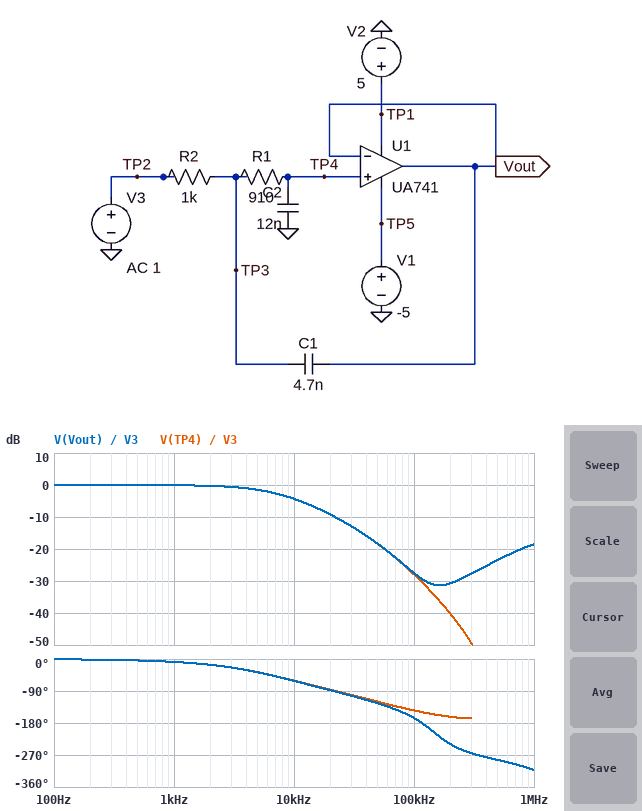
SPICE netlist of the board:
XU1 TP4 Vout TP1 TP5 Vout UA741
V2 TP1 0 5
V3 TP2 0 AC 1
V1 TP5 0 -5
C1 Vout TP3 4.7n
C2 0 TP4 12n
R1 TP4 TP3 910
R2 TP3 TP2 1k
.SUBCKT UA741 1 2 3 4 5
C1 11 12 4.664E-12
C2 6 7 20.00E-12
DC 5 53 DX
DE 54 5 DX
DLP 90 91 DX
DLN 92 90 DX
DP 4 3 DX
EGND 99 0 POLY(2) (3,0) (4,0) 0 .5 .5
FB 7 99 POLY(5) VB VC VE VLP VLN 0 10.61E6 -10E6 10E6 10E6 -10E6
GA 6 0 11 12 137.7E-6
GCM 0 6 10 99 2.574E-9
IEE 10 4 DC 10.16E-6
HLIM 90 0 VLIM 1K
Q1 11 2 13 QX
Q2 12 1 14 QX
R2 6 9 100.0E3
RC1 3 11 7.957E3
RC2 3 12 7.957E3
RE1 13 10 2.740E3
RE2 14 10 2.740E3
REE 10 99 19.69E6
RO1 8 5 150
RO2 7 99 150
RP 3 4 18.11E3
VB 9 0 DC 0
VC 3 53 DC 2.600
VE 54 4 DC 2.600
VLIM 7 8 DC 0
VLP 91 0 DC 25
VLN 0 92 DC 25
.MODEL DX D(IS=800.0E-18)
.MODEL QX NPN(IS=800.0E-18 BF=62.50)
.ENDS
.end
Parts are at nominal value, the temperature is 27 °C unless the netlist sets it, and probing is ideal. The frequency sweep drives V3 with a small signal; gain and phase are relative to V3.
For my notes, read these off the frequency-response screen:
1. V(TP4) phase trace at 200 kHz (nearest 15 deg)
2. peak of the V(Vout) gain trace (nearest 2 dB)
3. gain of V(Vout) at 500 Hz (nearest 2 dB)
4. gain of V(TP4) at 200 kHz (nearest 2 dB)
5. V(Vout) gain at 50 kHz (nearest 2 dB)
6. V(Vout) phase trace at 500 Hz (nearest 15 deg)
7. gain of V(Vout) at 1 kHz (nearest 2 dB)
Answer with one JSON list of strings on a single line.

["-165 deg", "0 dB", "0 dB", "-40 dB", "-18 dB", "0 deg", "0 dB"]
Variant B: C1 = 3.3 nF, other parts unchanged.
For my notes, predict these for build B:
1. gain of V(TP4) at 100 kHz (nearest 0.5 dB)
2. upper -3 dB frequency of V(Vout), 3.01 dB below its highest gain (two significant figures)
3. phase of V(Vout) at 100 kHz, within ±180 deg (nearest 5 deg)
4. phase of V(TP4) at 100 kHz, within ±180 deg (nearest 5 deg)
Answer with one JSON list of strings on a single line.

["-26.0 dB", "7.5 kHz", "-150 deg", "-135 deg"]
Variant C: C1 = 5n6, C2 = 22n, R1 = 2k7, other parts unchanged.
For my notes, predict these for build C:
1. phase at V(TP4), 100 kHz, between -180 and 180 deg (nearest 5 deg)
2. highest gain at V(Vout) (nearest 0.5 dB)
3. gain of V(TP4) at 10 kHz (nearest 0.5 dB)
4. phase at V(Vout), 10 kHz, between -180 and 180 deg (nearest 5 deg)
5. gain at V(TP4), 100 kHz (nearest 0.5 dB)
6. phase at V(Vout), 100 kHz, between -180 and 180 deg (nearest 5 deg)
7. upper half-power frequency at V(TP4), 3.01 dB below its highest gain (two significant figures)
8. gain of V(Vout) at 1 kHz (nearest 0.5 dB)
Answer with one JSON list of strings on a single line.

["-160 deg", "0 dB", "-14.0 dB", "-95 deg", "-43.5 dB", "135 deg", "2.1 kHz", "-1.0 dB"]
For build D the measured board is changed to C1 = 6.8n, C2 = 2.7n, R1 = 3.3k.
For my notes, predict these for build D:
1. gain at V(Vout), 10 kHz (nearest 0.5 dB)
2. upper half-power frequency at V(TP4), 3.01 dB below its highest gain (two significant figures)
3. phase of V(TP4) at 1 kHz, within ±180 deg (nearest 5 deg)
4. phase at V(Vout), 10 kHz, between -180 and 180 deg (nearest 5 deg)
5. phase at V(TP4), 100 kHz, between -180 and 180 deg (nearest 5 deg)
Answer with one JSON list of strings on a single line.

["-0.5 dB", "19 kHz", "-5 deg", "-45 deg", "-165 deg"]
